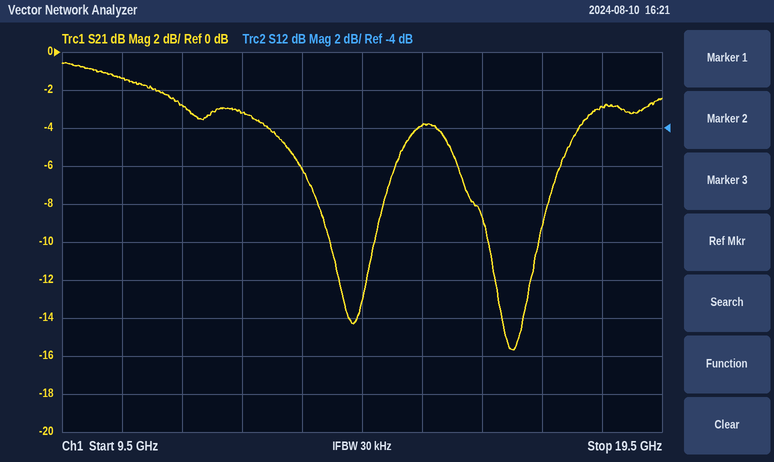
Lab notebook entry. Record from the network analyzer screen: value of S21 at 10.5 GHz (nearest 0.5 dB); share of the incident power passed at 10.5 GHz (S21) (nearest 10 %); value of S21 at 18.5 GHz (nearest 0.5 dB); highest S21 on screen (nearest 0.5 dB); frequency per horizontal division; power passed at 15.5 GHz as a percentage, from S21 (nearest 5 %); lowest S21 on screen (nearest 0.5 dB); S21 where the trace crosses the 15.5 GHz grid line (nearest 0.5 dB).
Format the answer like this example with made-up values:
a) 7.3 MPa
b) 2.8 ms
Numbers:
a) -1.5 dB
b) 70 %
c) -3.0 dB
d) -0.5 dB
e) 1 GHz
f) 40 %
g) -15.5 dB
h) -4.0 dB
